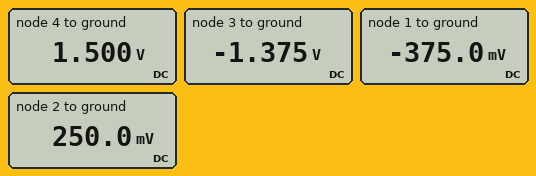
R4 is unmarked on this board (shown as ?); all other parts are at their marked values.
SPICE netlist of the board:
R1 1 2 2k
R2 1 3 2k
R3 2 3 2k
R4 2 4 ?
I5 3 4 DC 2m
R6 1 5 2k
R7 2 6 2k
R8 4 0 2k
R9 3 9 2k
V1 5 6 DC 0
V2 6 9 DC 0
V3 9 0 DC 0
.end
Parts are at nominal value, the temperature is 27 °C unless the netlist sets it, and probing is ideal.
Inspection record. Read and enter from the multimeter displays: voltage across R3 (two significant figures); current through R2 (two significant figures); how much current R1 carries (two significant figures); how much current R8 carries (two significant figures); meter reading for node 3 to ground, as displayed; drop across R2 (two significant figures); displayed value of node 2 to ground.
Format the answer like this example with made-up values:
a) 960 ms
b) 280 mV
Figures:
a) 1.6 V
b) 500 µA
c) 310 µA
d) 750 µA
e) -1.375 V
f) 1.0 V
g) 250.0 mV
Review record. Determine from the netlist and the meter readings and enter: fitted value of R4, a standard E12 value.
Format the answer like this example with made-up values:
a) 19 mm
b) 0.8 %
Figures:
a) 1 kΩ
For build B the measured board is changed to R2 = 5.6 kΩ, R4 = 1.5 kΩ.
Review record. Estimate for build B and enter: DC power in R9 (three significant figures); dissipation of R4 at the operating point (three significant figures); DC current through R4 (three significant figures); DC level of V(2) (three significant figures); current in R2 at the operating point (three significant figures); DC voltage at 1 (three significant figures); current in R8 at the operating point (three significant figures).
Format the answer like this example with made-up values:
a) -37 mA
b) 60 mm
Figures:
a) 1.41 mW
b) 1.85 mW
c) 1.11 mA
d) 111 mV
e) 263 µA
f) -208 mV
g) 889 µA
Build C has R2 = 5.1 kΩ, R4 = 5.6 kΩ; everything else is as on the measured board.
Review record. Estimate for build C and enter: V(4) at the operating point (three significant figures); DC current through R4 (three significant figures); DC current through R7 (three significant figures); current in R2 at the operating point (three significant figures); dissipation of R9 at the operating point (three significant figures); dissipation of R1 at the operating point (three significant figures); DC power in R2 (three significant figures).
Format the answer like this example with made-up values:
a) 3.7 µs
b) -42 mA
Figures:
a) 2.84 V
b) 581 µA
c) 209 µA
d) 282 µA
e) 1.86 mW
f) 2.62 µW
g) 405 µW
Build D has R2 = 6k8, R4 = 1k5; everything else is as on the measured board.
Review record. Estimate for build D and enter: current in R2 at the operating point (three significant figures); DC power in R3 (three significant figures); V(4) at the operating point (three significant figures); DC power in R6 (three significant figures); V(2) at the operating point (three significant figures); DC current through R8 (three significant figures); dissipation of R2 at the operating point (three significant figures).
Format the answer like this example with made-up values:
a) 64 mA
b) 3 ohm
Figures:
a) 227 µA
b) 1.67 mW
c) 1.78 V
d) 14.7 µW
e) 111 mV
f) 889 µA
g) 351 µW
